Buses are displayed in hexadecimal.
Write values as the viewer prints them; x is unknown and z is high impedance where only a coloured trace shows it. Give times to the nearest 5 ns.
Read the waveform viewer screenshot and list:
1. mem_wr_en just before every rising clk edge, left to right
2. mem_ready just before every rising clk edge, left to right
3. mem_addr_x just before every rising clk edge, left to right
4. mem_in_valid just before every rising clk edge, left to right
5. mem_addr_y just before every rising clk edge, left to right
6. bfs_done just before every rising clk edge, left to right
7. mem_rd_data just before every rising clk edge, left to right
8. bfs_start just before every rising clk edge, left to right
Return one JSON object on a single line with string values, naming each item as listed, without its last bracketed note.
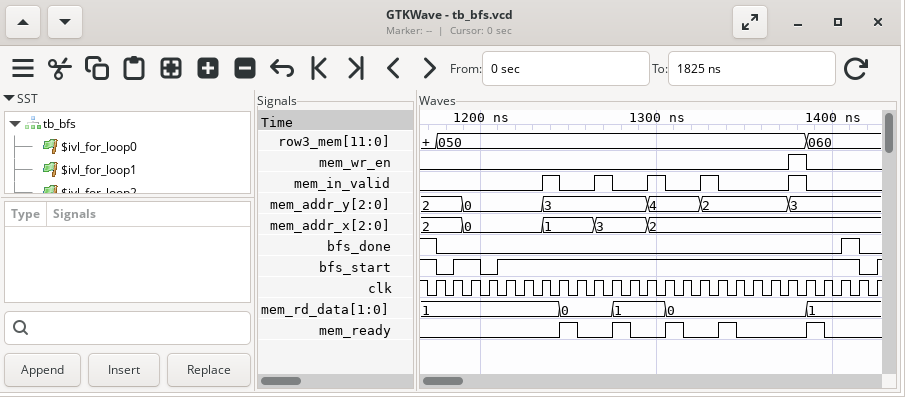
{"mem_wr_en just before every rising clk edge, left to right": "0 0 0 0 0 0 0 0 0 0 0 0 0 0 0 0 0 0 0 0 0 1 0 0 0 0", "mem_ready just before every rising clk edge, left to right": "0 0 0 0 0 0 0 0 1 0 0 1 0 0 1 0 0 1 0 0 0 0 1 0 0 0", "mem_addr_x just before every rising clk edge, left to right": "2, 2, 0, 0, 0, 0, 0, 1, 1, 1, 3, 3, 3, 2, 2, 2, 2, 2, 2, 2, 2, 2, 2, 2, 2, 2", "mem_in_valid just before every rising clk edge, left to right": "0 0 0 0 0 0 0 1 0 0 1 0 0 1 0 0 1 0 0 0 0 1 0 0 0 0", "mem_addr_y just before every rising clk edge, left to right": "2, 2, 0, 0, 0, 0, 0, 3, 3, 3, 3, 3, 3, 4, 4, 4, 2, 2, 2, 2, 2, 3, 3, 3, 3, 3", "bfs_done just before every rising clk edge, left to right": "1 0 0 0 0 0 0 0 0 0 0 0 0 0 0 0 0 0 0 0 0 0 0 0 1 0", "mem_rd_data just before every rising clk edge, left to right": "1, 1, 1, 1, 1, 1, 1, 1, 0, 0, 0, 1, 1, 1, 0, 0, 0, 0, 0, 0, 0, 0, 1, 1, 1, 1", "bfs_start just before every rising clk edge, left to right": "1 0 1 0 1 1 1 1 1 1 1 1 1 1 1 1 1 1 1 1 1 1 1 1 1 0"}
